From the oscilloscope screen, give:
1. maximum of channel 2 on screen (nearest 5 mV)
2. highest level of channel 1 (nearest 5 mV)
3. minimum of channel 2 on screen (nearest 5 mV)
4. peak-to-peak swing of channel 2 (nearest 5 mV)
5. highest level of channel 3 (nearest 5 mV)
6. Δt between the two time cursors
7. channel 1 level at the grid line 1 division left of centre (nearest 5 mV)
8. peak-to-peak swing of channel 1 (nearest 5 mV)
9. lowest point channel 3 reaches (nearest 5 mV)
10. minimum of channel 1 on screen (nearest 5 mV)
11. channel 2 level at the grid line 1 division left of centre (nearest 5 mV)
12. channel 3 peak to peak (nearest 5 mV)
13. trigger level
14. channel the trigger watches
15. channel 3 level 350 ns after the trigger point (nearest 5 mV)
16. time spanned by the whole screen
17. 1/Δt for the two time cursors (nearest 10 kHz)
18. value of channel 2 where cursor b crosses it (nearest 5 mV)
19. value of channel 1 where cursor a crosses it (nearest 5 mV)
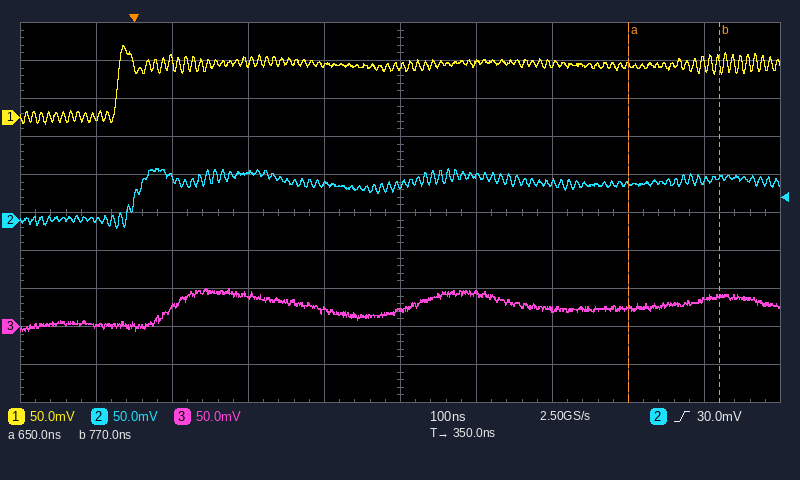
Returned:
70 mV
95 mV
-10 mV
80 mV
50 mV
120 ns
70 mV
105 mV
-5 mV
-10 mV
45 mV
55 mV
30.0 mV
channel 2
20 mV
1 µs
8.33 MHz
55 mV
70 mV
